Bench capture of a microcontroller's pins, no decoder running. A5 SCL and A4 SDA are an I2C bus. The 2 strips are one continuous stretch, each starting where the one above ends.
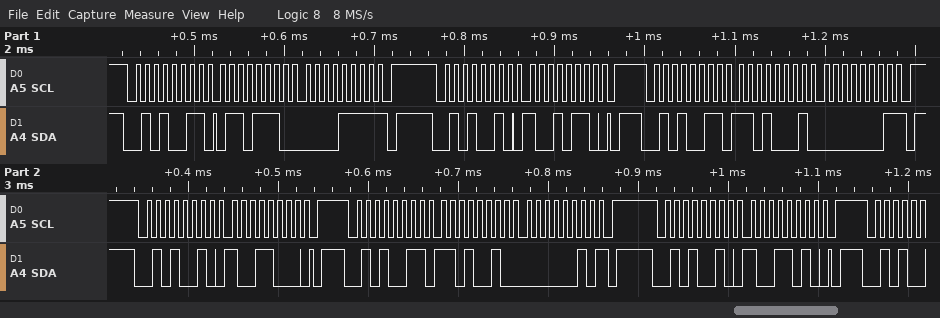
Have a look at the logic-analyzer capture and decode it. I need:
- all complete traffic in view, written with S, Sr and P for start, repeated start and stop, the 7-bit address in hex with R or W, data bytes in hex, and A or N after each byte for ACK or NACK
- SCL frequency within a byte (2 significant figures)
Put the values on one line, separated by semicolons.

S 29R A 6E A 0F N P S 29W A 96 A P S 29R A D1 A 01 N P S 29W A 98 A P S 29R A D2 A 02 N P S 29W A 9A A P; 100 kHz
